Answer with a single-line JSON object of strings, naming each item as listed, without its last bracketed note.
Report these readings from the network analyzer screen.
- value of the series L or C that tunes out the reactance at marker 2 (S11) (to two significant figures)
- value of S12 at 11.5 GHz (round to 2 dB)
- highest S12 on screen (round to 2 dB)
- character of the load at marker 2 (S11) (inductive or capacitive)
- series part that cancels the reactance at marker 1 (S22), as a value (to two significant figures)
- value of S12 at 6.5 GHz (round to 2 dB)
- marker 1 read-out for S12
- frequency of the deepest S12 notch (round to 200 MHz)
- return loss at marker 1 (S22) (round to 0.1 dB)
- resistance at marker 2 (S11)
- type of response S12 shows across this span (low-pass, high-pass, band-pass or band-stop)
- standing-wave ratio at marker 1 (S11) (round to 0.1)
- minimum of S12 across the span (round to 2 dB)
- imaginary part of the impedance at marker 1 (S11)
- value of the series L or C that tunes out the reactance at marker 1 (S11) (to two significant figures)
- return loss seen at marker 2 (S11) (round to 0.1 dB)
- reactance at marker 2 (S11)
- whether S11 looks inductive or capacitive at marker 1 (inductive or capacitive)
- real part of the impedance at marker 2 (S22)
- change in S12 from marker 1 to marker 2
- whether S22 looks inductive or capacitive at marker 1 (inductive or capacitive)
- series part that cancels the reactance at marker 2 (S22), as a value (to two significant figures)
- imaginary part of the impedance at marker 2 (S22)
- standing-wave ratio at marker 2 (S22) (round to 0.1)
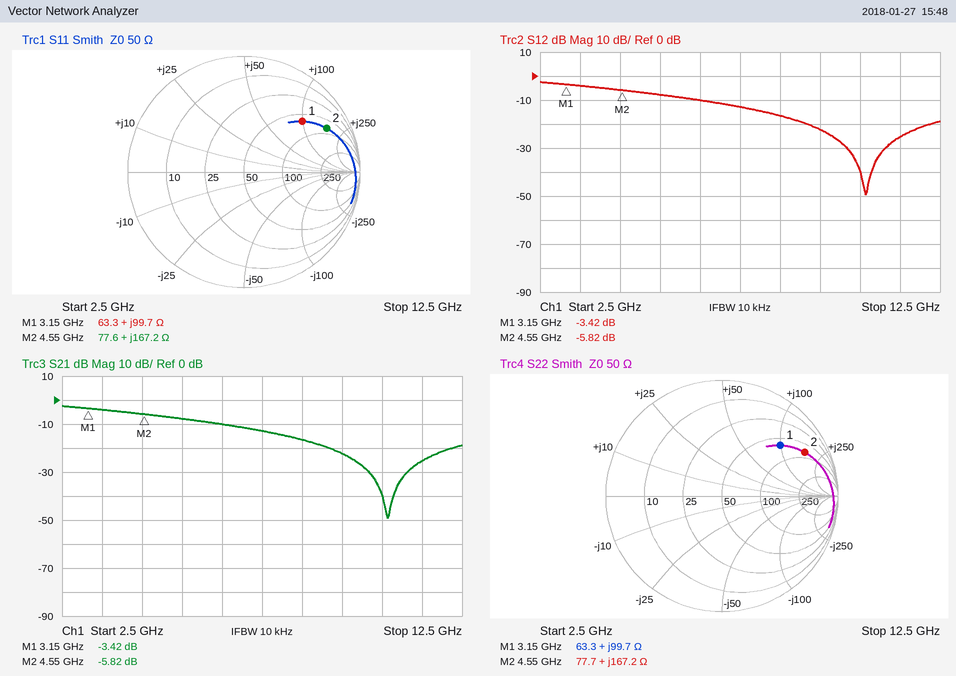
{"value of the series L or C that tunes out the reactance at marker 2 (S11)": "210 fF", "value of S12 at 11.5 GHz": "-26 dB", "highest S12 on screen": "-2 dB", "character of the load at marker 2 (S11)": "inductive", "series part that cancels the reactance at marker 1 (S22), as a value": "510 fF", "value of S12 at 6.5 GHz": "-10 dB", "marker 1 read-out for S12": "-3.42 dB", "frequency of the deepest S12 notch": "10.6 GHz", "return loss at marker 1 (S22)": "3.5 dB", "resistance at marker 2": "77.6 Ω", "type of response S12 shows across this span": "low-pass", "standing-wave ratio at marker 1 (S11)": "5.0", "minimum of S12 across the span": "-50 dB", "imaginary part of the impedance at marker 1": "+99.7 Ω", "value of the series L or C that tunes out the reactance at marker 1 (S11)": "510 fF", "return loss seen at marker 2 (S11)": "1.9 dB", "reactance at marker 2": "+167.2 Ω", "whether S11 looks inductive or capacitive at marker 1": "inductive", "real part of the impedance at marker 2": "77.7 Ω", "change in S12 from marker 1 to marker 2": "-2.40 dB", "whether S22 looks inductive or capacitive at marker 1": "inductive", "series part that cancels the reactance at marker 2 (S22), as a value": "210 fF", "imaginary part of the impedance at marker 2": "+167.2 Ω", "standing-wave ratio at marker 2 (S22)": "9.3"}
